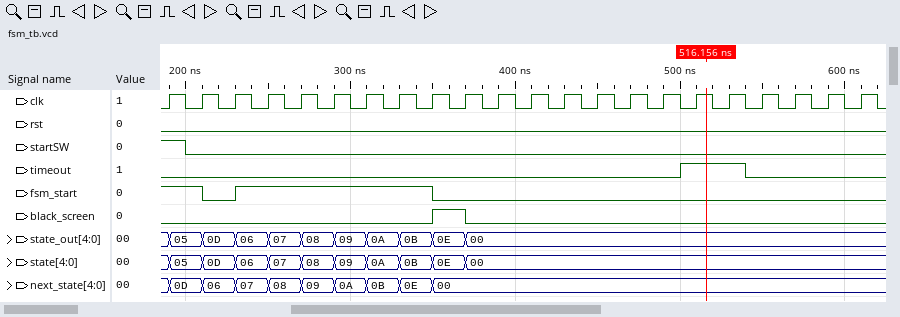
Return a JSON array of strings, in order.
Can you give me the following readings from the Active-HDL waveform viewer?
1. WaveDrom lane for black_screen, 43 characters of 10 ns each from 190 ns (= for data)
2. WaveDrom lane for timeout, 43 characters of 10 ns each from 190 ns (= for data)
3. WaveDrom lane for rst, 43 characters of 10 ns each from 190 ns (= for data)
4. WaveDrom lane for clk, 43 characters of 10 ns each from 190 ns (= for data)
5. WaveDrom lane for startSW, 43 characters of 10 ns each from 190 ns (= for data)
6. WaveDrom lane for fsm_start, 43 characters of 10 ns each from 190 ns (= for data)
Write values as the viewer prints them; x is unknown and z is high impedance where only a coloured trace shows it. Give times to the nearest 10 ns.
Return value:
["{name: 'black_screen', wave: '0...............1.0........................'}", "{name: 'timeout', wave: '0..............................1...0.......'}", "{name: 'rst', wave: '0..........................................'}", "{name: 'clk', wave: '1010101010101010101010101010101010101010101'}", "{name: 'startSW', wave: '10.........................................'}", "{name: 'fsm_start', wave: '1.0.1...........0..........................'}"]
